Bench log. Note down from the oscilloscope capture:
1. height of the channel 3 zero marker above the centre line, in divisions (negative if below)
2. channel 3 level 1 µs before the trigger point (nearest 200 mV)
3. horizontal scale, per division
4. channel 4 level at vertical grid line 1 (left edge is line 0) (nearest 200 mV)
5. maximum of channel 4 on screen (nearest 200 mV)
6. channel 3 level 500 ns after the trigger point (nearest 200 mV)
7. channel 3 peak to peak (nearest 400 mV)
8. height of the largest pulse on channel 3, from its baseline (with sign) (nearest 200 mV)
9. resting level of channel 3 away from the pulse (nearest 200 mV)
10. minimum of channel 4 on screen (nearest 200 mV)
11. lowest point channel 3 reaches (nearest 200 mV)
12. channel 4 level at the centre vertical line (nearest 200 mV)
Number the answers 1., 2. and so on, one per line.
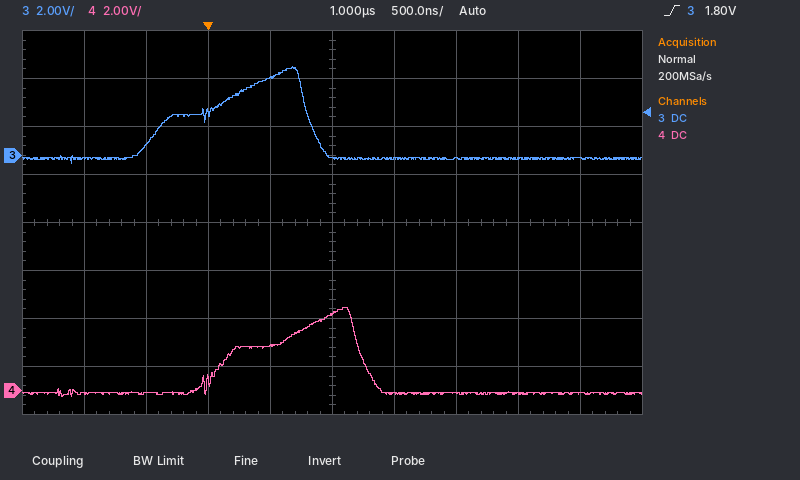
1. +1.4 div
2. -200 mV
3. 500 ns
4. -200 mV
5. 3.4 V
6. 3.2 V
7. 4.0 V
8. +3.8 V
9. -200 mV
10. -200 mV
11. -400 mV
12. 3.2 V
